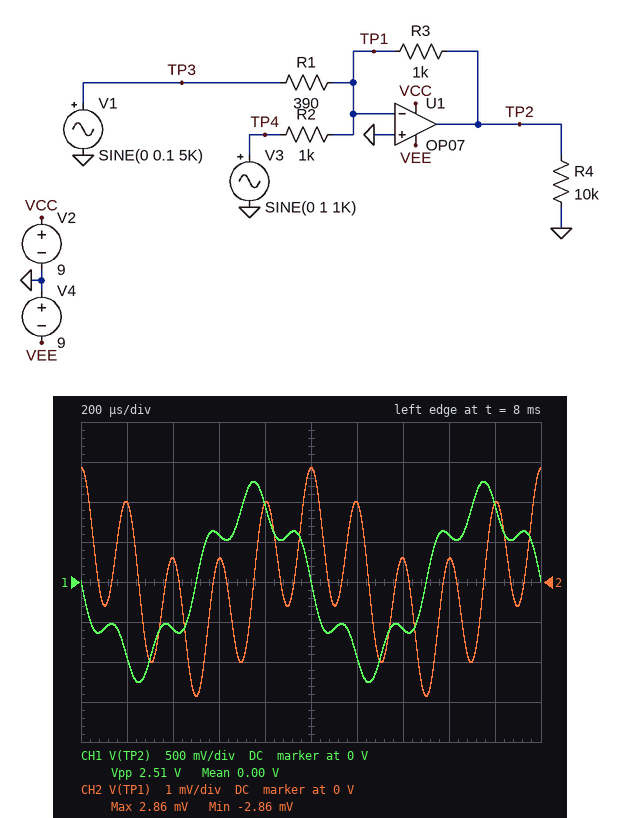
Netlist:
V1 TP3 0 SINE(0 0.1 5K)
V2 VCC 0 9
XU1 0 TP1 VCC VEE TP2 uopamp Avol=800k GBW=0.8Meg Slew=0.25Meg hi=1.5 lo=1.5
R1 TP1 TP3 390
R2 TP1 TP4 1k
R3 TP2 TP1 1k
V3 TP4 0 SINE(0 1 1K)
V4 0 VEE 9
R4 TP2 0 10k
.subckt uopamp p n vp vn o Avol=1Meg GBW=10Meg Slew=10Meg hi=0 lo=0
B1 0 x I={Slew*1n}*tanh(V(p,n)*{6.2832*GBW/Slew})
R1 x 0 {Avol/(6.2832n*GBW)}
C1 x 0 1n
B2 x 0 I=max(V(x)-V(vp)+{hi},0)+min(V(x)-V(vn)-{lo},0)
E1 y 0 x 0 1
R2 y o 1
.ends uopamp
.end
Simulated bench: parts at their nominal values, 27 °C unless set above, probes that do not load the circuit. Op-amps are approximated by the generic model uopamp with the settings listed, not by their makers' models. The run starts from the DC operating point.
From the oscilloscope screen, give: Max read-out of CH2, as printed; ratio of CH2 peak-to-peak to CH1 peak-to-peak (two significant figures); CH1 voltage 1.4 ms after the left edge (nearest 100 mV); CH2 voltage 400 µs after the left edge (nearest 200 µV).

2.86 mV
0.0023
-600 mV
600 µV
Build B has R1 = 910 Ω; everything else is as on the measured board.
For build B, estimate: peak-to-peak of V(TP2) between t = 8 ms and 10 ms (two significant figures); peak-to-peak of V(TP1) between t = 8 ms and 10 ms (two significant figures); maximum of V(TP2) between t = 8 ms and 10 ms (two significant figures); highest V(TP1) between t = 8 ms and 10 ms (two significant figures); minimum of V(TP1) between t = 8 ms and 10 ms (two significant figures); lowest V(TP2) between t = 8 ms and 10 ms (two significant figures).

2.2 V
3.9 mV
1.1 V
1.9 mV
-1.9 mV
-1.1 V
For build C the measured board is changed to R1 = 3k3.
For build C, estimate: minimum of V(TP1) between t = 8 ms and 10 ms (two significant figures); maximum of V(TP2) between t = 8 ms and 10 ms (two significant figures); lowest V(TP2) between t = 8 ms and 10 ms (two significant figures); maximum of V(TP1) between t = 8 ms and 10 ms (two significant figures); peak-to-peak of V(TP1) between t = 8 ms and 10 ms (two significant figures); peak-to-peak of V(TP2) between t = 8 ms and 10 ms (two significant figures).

-1.4 mV
1.0 V
-1.0 V
1.4 mV
2.9 mV
2.1 V
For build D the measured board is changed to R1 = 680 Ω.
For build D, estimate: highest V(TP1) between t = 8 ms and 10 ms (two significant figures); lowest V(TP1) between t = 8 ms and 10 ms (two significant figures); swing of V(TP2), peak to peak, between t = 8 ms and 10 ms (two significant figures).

2.2 mV
-2.2 mV
2.3 V
